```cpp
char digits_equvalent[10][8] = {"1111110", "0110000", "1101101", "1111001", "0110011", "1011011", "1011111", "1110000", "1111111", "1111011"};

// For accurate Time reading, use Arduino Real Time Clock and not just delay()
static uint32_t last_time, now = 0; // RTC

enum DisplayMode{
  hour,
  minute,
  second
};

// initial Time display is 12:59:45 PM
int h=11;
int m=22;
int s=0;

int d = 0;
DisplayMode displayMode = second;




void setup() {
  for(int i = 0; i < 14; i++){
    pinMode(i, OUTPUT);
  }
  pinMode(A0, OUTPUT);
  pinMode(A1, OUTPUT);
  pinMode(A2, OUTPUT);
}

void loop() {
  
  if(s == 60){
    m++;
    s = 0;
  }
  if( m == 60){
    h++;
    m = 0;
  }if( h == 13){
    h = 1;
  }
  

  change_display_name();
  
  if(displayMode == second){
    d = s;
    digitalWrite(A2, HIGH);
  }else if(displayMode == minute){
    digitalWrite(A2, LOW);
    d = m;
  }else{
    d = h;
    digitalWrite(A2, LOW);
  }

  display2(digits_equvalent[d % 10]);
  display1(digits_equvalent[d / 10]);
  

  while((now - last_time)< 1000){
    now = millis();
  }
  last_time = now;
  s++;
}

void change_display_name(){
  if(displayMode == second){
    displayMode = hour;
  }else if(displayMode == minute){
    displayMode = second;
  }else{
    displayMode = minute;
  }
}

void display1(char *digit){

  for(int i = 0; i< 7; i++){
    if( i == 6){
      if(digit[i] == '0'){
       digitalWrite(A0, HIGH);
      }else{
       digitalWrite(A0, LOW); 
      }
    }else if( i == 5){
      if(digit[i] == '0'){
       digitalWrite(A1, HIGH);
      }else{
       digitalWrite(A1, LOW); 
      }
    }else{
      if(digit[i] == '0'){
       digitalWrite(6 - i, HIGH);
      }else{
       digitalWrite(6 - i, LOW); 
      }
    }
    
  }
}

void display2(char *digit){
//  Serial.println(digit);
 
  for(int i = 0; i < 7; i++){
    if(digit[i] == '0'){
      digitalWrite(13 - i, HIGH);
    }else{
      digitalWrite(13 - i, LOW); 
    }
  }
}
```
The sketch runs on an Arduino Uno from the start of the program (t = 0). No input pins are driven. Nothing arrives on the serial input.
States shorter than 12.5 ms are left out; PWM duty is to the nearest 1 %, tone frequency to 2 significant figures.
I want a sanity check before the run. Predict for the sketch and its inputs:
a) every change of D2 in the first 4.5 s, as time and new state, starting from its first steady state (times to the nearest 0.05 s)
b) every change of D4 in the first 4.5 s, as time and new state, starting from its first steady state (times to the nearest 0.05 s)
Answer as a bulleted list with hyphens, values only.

- 0 s high; 1 s low; 3 s high; 4 s low
- 0 s low; 1 s high; 2 s low; 4 s high
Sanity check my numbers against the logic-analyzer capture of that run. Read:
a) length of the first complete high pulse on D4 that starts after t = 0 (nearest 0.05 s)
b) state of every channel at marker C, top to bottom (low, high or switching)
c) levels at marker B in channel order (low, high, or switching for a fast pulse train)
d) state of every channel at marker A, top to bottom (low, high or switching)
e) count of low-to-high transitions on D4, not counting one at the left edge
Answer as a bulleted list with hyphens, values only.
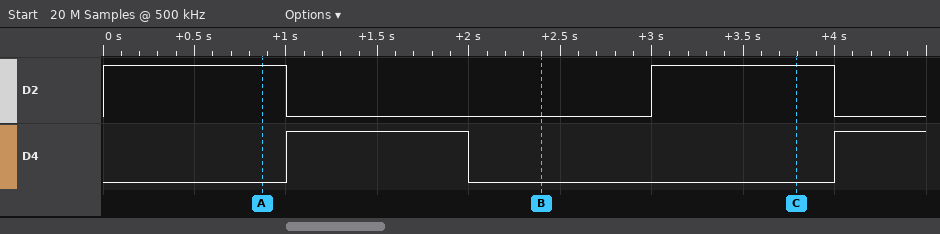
- 1.00 s
- D2 high, D4 low
- D2 low, D4 low
- D2 high, D4 low
- 2
